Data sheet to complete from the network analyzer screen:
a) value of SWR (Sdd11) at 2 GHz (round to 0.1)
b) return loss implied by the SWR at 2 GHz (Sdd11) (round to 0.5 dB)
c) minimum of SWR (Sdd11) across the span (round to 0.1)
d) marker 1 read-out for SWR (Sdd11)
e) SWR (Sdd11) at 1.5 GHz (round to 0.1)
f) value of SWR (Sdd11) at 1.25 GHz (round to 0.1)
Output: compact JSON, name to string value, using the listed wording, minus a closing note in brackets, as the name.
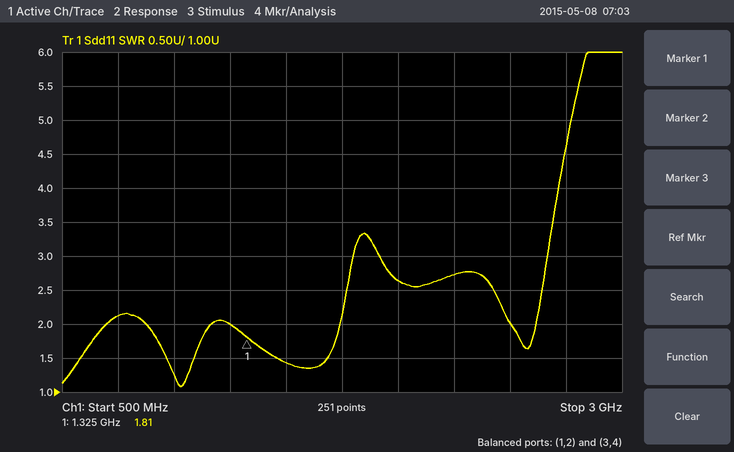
{"value of SWR (Sdd11) at 2 GHz": "2.6", "return loss implied by the SWR at 2 GHz (Sdd11)": "7.0 dB", "minimum of SWR (Sdd11) across the span": "1.1", "marker 1 read-out for SWR": "1.81", "SWR (Sdd11) at 1.5 GHz": "1.4", "value of SWR (Sdd11) at 1.25 GHz": "2.0"}
